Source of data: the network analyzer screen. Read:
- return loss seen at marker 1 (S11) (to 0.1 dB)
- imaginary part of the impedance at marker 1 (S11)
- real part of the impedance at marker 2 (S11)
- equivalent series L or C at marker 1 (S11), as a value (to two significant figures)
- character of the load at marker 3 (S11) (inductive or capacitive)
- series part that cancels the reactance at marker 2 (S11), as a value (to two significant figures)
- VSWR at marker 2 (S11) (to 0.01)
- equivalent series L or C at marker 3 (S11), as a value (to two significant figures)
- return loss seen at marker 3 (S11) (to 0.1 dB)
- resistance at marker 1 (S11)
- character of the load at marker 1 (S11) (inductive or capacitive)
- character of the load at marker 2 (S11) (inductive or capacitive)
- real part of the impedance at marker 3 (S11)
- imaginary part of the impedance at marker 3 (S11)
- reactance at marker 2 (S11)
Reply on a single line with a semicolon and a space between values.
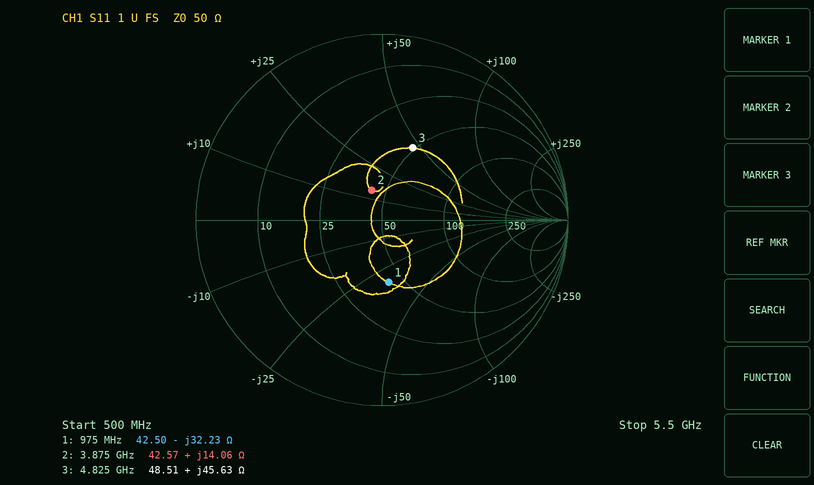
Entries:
9.4 dB; -32.23 Ω; 42.57 Ω; 5.1 pF; inductive; 2.9 pF; 1.41; 1.5 nH; 7.5 dB; 42.50 Ω; capacitive; inductive; 48.51 Ω; +45.63 Ω; +14.06 Ω
